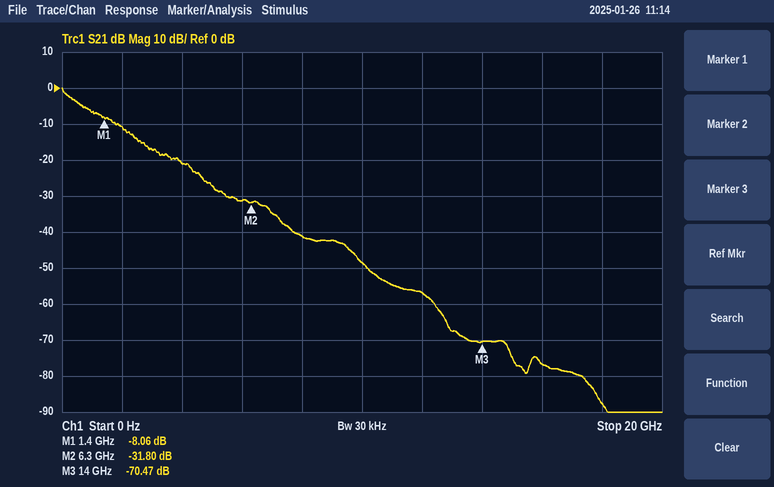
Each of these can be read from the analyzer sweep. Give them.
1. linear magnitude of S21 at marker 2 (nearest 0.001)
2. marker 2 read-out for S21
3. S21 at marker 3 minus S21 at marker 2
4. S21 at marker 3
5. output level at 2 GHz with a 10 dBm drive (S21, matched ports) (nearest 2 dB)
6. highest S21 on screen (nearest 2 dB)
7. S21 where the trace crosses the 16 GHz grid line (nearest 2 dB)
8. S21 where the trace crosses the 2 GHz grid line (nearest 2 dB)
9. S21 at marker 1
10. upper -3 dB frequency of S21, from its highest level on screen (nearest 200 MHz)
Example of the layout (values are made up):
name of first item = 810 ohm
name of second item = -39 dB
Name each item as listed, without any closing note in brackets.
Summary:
linear magnitude of S21 at marker 2 = 0.026
marker 2 read-out for S21 = -31.80 dB
S21 at marker 3 minus S21 at marker 2 = -38.67 dB
S21 at marker 3 = -70.47 dB
output level at 2 GHz with a 10 dBm drive (S21, matched ports) = 0 dBm
highest S21 on screen = 0 dB
S21 where the trace crosses the 16 GHz grid line = -76 dB
S21 where the trace crosses the 2 GHz grid line = -10 dB
S21 at marker 1 = -8.06 dB
upper -3 dB frequency of S21, from its highest level on screen = 400 MHz
